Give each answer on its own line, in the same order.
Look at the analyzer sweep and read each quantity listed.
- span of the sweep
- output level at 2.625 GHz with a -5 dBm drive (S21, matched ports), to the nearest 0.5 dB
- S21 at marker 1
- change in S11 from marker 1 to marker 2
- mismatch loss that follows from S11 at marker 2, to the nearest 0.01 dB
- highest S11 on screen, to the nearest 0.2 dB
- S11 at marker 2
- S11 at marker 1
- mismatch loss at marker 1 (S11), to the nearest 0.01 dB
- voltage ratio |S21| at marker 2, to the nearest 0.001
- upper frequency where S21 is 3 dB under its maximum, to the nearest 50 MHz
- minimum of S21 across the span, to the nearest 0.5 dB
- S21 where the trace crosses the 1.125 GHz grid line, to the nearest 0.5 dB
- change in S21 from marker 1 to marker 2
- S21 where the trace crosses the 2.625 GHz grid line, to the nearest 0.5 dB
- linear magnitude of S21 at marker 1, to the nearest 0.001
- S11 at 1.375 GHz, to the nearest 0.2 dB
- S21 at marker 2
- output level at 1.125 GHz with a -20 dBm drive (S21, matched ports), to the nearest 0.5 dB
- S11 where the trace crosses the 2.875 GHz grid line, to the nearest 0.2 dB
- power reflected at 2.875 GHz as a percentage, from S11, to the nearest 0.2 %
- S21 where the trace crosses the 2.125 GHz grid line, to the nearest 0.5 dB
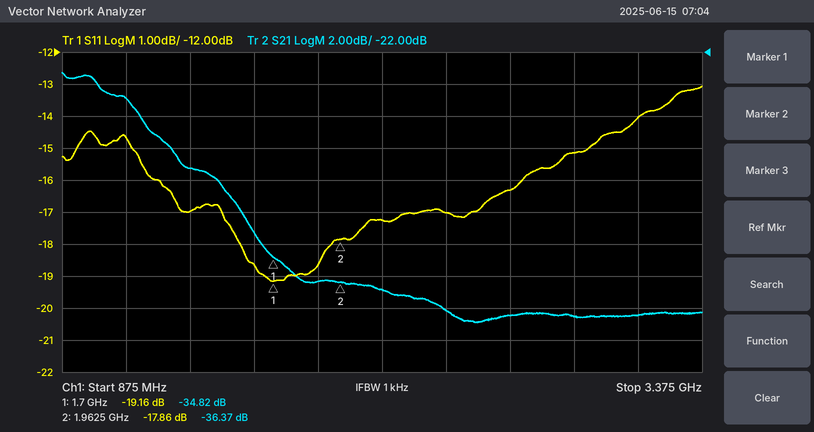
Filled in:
2.5 GHz
-43.5 dBm
-34.82 dB
1.30 dB
0.07 dB
-13.0 dB
-17.86 dB
-19.16 dB
0.05 dB
0.015
1.20 GHz
-39.0 dB
-25.0 dB
-1.55 dB
-38.5 dB
0.018
-17.0 dB
-36.37 dB
-45.0 dBm
-15.2 dB
3.0 %
-37.0 dB
